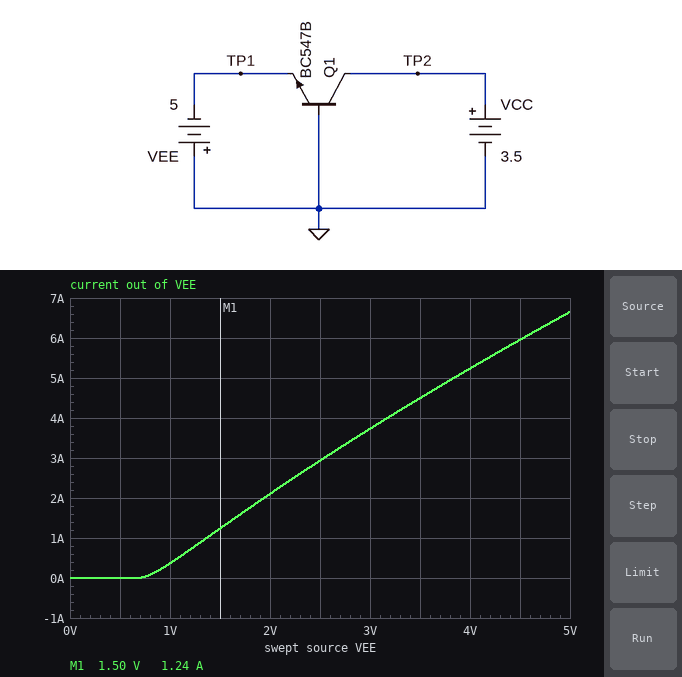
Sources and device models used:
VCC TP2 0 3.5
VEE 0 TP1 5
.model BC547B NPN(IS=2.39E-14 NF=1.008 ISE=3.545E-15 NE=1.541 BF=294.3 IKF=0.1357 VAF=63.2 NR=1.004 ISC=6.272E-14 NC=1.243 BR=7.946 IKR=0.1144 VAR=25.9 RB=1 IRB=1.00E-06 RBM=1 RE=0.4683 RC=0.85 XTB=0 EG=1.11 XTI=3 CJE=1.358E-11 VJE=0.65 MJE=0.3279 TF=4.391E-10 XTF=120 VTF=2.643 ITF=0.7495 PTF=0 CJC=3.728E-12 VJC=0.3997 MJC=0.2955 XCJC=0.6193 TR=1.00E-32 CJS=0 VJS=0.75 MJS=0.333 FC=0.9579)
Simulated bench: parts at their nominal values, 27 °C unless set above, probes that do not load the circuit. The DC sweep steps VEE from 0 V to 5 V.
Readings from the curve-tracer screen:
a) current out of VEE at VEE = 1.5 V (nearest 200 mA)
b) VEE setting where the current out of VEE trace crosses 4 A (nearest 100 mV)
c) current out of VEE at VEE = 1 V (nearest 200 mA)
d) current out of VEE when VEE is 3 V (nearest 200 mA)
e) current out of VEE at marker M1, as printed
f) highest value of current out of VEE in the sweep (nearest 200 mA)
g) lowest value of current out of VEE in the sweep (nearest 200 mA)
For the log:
1.2 A
3.2 V
400 mA
3.8 A
1.24 A
6.6 A
0 A
